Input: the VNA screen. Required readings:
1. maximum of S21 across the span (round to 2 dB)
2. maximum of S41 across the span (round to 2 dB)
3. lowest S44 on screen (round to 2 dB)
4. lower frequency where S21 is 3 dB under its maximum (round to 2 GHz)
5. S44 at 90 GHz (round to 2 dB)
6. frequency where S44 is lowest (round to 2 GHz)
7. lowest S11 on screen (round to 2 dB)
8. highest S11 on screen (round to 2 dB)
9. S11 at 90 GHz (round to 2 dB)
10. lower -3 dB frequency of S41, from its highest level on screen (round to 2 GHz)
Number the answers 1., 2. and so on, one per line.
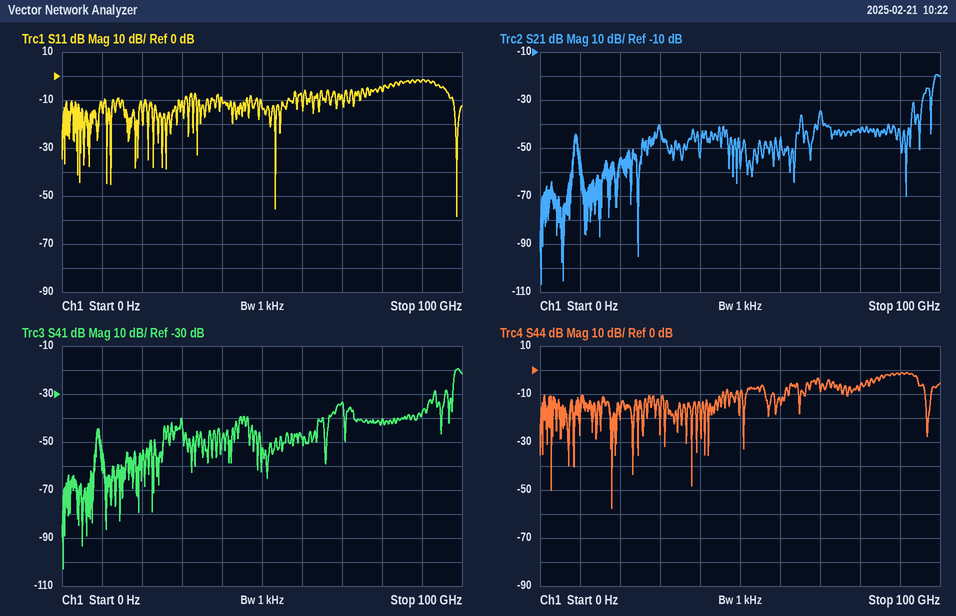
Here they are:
1. -20 dB
2. -20 dB
3. -58 dB
4. 98 GHz
5. -2 dB
6. 18 GHz
7. -58 dB
8. -2 dB
9. -2 dB
10. 98 GHz
